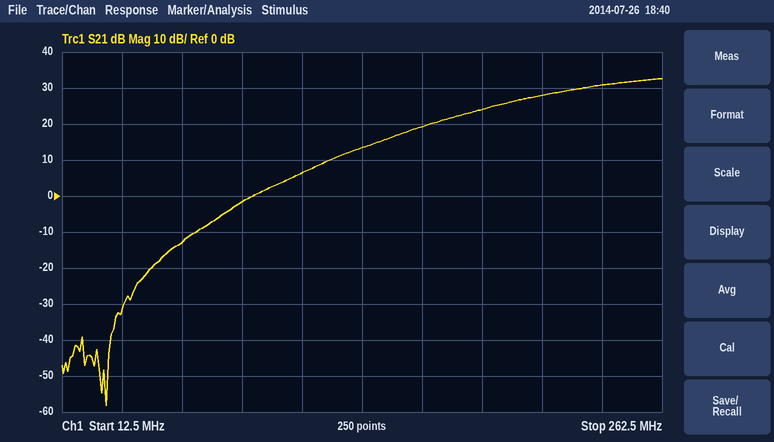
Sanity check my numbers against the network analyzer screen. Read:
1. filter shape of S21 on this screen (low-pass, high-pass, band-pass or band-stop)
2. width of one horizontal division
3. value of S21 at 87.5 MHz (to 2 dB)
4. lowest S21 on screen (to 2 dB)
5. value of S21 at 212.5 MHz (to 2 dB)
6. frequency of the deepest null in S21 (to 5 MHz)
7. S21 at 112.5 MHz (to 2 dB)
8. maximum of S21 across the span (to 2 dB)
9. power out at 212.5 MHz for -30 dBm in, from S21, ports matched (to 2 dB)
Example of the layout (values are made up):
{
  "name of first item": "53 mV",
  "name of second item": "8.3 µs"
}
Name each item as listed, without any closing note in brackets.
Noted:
{
  "filter shape of S21 on this screen": "high-pass",
  "width of one horizontal division": "25 MHz",
  "value of S21 at 87.5 MHz": "-2 dB",
  "lowest S21 on screen": "-58 dB",
  "value of S21 at 212.5 MHz": "28 dB",
  "frequency of the deepest null in S21": "30 MHz",
  "S21 at 112.5 MHz": "6 dB",
  "maximum of S21 across the span": "32 dB",
  "power out at 212.5 MHz for -30 dBm in, from S21, ports matched": "-2 dBm"
}
